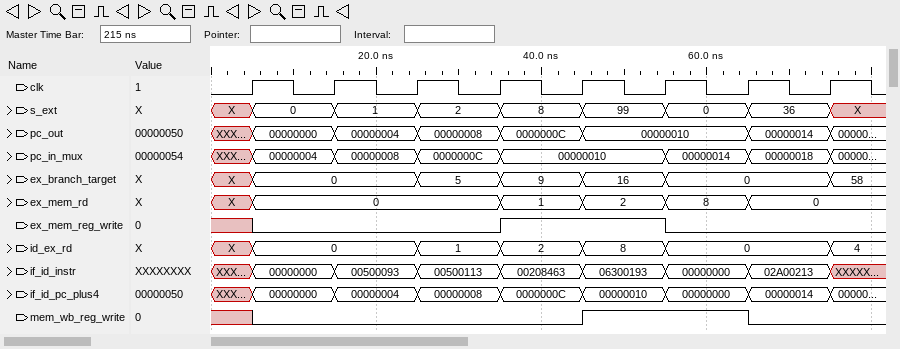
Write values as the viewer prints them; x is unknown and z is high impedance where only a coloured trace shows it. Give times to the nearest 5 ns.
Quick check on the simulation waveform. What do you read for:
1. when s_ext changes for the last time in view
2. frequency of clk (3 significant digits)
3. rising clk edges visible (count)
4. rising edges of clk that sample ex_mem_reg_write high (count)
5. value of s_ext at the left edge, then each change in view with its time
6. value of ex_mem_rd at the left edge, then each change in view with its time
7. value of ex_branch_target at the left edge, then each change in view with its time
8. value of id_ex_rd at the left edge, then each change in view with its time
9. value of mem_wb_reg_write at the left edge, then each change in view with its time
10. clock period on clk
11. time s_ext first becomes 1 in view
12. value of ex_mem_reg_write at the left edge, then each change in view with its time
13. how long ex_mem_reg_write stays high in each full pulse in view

75 ns
100 MHz
8
2
X, 0 at 5 ns, 1 at 15 ns, 2 at 25 ns, 8 at 35 ns, 99 at 45 ns, 0 at 55 ns, 36 at 65 ns, X at 75 ns
X, 0 at 5 ns, 1 at 35 ns, 2 at 45 ns, 8 at 55 ns, 0 at 65 ns
X, 0 at 5 ns, 5 at 25 ns, 9 at 35 ns, 16 at 45 ns, 0 at 55 ns, 58 at 75 ns
X, 0 at 5 ns, 1 at 25 ns, 2 at 35 ns, 8 at 45 ns, 0 at 55 ns, 4 at 75 ns
x, 0 at 5 ns, 1 at 45 ns, 0 at 65 ns
10 ns
15 ns
x, 0 at 5 ns, 1 at 35 ns, 0 at 55 ns
20 ns
